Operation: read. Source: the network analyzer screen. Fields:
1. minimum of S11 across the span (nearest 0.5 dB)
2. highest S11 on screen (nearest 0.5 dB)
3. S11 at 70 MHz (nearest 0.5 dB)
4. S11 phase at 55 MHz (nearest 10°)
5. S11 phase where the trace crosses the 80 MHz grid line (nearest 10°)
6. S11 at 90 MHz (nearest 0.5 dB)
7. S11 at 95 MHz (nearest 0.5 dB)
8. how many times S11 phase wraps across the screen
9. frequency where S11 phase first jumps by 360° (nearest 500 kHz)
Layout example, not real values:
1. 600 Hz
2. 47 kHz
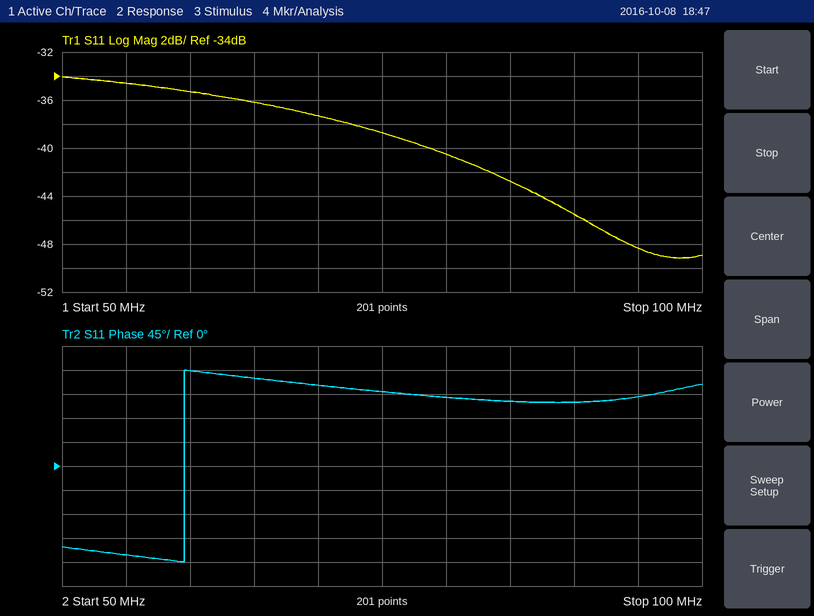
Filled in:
1. -49.0 dB
2. -34.0 dB
3. -37.5 dB
4. -170°
5. 130°
6. -45.5 dB
7. -48.5 dB
8. 1
9. 59.5 MHz
